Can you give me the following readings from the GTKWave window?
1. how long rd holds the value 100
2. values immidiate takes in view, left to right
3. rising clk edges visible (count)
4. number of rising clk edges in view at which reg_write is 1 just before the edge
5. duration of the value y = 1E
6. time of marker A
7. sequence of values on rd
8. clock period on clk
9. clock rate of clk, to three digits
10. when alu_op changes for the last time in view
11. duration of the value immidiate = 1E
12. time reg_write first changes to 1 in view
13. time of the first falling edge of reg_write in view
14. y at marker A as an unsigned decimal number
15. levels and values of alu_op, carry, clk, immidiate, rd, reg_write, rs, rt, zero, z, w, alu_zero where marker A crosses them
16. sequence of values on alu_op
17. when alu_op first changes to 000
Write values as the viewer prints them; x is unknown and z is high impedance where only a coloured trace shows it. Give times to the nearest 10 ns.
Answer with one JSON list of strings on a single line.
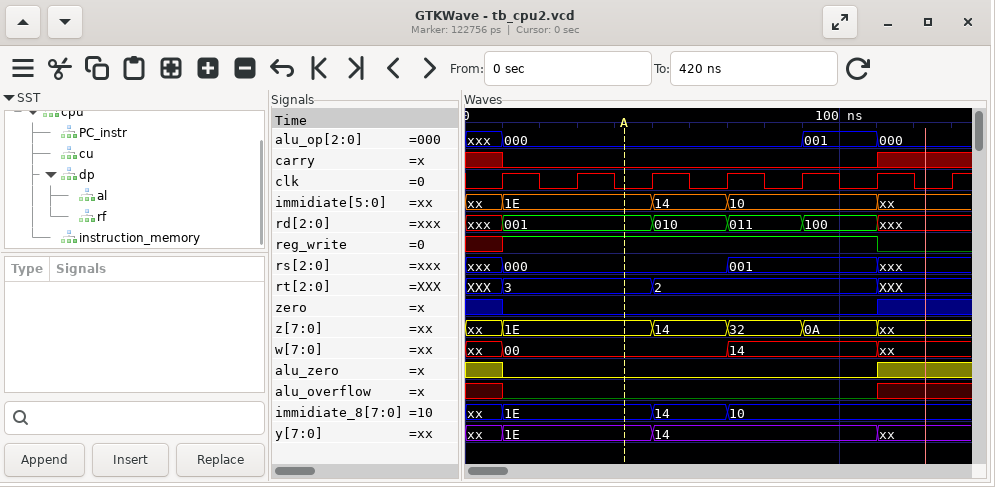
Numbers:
["20 ns", "xx, 1E, 14, 10, xx", "7", "5", "40 ns", "40 ns", "xxx, 001, 010, 011, 100, xxx", "20 ns", "50.0 MHz", "110 ns", "40 ns", "10 ns", "110 ns", "30", "alu_op=000, carry=0, clk=0, immidiate=1E, rd=001, reg_write=1, rs=000, rt=3, zero=0, z=1E, w=00, alu_zero=0", "xxx, 000, 001, 000", "10 ns"]
